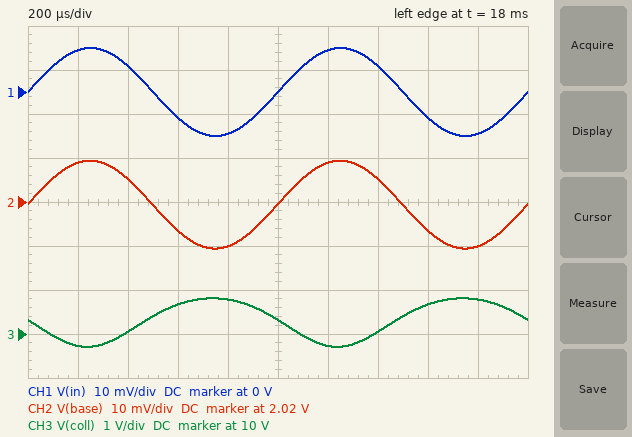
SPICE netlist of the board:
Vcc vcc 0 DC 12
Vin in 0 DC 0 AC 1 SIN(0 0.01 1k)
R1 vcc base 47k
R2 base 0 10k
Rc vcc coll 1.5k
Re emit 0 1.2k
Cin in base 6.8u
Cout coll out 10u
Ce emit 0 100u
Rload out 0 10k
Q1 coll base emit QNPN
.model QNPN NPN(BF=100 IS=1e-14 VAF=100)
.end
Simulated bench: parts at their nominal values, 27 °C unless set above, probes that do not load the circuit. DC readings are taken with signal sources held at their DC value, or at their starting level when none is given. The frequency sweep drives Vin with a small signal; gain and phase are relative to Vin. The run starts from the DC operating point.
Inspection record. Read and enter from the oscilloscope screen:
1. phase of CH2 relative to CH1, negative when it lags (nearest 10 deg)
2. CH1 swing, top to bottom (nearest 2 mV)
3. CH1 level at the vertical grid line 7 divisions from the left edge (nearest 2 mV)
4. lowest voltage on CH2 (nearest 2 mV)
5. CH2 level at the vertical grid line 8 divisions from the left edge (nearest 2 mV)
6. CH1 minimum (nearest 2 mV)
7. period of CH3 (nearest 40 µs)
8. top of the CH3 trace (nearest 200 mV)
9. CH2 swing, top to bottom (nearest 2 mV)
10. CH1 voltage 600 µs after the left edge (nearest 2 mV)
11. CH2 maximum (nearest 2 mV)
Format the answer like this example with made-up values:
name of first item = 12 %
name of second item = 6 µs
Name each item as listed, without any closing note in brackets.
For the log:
phase of CH2 relative to CH1, negative when it lags = 0 deg
CH1 swing, top to bottom = 20 mV
CH1 level at the vertical grid line 7 divisions from the left edge = 6 mV
lowest voltage on CH2 = 2.010 V
CH2 level at the vertical grid line 8 divisions from the left edge = 2.014 V
CH1 minimum = -10 mV
period of CH3 = 1.00 ms
top of the CH3 trace = 10.8 V
CH2 swing, top to bottom = 20 mV
CH1 voltage 600 µs after the left edge = -6 mV
CH2 maximum = 2.030 V
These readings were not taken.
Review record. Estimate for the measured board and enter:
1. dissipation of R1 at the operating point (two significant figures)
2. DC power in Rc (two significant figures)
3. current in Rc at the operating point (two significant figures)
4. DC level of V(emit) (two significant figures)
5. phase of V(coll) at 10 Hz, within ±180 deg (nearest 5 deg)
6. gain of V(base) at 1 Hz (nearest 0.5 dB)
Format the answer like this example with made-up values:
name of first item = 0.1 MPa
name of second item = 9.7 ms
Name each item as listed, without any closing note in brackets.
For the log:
dissipation of R1 at the operating point = 2.1 mW
DC power in Rc = 1.9 mW
current in Rc at the operating point = 1.1 mA
DC level of V(emit) = 1.4 V
phase of V(coll) at 10 Hz, within ±180 deg = -90 deg
gain of V(base) at 1 Hz = -10.0 dB
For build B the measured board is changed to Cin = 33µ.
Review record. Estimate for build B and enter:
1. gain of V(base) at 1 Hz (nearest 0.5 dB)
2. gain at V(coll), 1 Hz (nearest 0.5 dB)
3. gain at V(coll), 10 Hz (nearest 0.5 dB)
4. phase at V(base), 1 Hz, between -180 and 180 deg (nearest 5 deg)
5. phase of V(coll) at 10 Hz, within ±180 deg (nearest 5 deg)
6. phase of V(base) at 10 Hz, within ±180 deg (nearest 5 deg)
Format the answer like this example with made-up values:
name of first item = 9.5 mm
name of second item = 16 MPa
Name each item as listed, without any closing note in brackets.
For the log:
gain of V(base) at 1 Hz = -1.5 dB
gain at V(coll), 1 Hz = 1.5 dB
gain at V(coll), 10 Hz = 18.0 dB
phase at V(base), 1 Hz, between -180 and 180 deg = 30 deg
phase of V(coll) at 10 Hz, within ±180 deg = -105 deg
phase of V(base) at 10 Hz, within ±180 deg = 5 deg
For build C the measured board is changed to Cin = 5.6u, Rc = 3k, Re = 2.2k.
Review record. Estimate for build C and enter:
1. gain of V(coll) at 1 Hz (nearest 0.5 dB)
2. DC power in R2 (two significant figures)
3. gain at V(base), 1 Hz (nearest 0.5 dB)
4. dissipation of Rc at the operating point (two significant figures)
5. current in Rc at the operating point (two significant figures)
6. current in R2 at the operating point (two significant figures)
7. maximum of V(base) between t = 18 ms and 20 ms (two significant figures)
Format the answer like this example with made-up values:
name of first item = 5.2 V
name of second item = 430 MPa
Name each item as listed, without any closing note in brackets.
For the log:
gain of V(coll) at 1 Hz = -5.0 dB
DC power in R2 = 420 µW
gain at V(base), 1 Hz = -11.5 dB
dissipation of Rc at the operating point = 1.2 mW
current in Rc at the operating point = 640 µA
current in R2 at the operating point = 210 µA
maximum of V(base) between t = 18 ms and 20 ms = 2.1 V
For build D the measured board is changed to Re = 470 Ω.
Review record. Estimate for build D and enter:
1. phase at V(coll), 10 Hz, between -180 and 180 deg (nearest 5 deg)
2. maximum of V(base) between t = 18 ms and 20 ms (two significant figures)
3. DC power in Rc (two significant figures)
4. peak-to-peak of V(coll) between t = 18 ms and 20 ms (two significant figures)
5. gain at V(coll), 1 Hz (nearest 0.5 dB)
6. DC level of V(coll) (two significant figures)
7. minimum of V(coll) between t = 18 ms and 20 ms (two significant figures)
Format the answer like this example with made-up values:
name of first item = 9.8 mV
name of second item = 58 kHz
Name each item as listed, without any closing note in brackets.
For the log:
phase at V(coll), 10 Hz, between -180 and 180 deg = -95 deg
maximum of V(base) between t = 18 ms and 20 ms = 1.9 V
DC power in Rc = 10 mW
peak-to-peak of V(coll) between t = 18 ms and 20 ms = 2.5 V
gain at V(coll), 1 Hz = -1.0 dB
DC level of V(coll) = 8.1 V
minimum of V(coll) between t = 18 ms and 20 ms = 6.8 V
